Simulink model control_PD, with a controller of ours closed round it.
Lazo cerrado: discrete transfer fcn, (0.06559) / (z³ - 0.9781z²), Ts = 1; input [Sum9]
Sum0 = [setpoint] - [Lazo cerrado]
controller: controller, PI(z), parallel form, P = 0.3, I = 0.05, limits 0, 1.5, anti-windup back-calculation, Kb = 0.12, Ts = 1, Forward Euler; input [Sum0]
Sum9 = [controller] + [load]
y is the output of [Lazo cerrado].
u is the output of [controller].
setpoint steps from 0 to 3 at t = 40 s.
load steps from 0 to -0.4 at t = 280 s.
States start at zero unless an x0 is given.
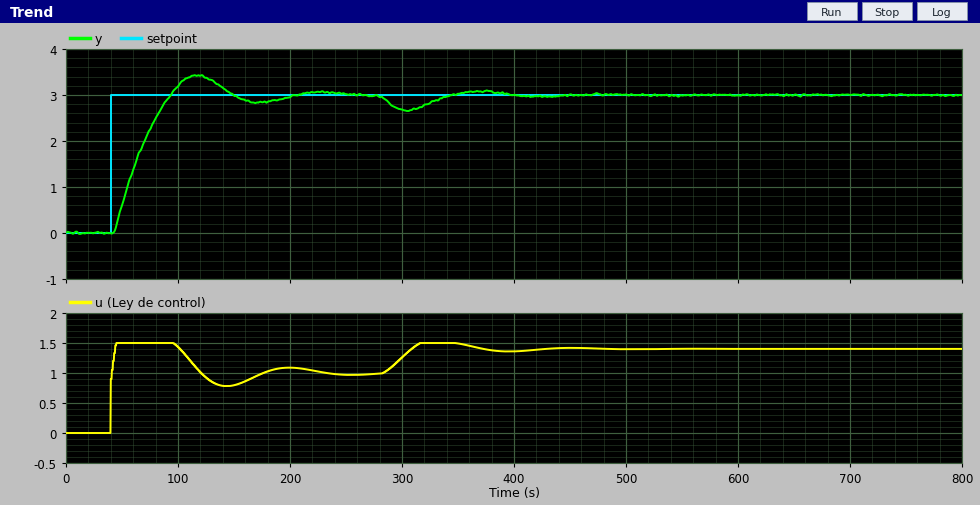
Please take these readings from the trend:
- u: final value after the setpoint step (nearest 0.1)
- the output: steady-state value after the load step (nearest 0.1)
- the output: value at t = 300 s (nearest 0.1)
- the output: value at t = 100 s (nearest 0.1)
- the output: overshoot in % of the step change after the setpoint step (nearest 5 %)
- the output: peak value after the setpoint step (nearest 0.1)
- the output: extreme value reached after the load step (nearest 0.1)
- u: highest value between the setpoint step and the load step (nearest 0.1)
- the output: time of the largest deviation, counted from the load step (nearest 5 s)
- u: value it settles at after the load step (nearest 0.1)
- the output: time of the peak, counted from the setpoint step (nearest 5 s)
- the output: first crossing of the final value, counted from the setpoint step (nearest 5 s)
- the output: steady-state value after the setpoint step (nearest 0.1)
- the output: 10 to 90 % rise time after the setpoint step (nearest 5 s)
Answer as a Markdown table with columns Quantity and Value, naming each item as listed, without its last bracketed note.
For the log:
| Quantity | Value |
|---|---|
| u: final value after the setpoint step | 1.0 |
| the output: steady-state value after the load step | 3.0 |
| the output: value at t = 300 s | 2.7 |
| the output: value at t = 100 s | 3.2 |
| the output: overshoot in % of the step change after the setpoint step | 15 % |
| the output: peak value after the setpoint step | 3.4 |
| the output: extreme value reached after the load step | 2.7 |
| u: highest value between the setpoint step and the load step | 1.5 |
| the output: time of the largest deviation, counted from the load step | 25 s |
| u: value it settles at after the load step | 1.4 |
| the output: time of the peak, counted from the setpoint step | 75 s |
| the output: first crossing of the final value, counted from the setpoint step | 55 s |
| the output: steady-state value after the setpoint step | 3.0 |
| the output: 10 to 90 % rise time after the setpoint step | 40 s |
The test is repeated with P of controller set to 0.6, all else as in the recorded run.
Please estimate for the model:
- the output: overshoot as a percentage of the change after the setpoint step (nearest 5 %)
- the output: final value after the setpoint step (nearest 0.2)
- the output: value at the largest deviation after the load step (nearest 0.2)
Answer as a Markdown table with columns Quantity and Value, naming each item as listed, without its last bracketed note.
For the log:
| Quantity | Value |
|---|---|
| the output: overshoot as a percentage of the change after the setpoint step | 10 % |
| the output: final value after the setpoint step | 3.0 |
| the output: value at the largest deviation after the load step | 2.8 |
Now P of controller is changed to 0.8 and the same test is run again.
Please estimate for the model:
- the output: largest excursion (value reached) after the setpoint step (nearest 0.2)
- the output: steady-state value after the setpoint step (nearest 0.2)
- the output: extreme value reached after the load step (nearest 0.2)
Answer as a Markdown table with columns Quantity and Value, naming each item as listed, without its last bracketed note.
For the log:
| Quantity | Value |
|---|---|
| the output: largest excursion (value reached) after the setpoint step | 3.2 |
| the output: steady-state value after the setpoint step | 3.0 |
| the output: extreme value reached after the load step | 2.8 |
